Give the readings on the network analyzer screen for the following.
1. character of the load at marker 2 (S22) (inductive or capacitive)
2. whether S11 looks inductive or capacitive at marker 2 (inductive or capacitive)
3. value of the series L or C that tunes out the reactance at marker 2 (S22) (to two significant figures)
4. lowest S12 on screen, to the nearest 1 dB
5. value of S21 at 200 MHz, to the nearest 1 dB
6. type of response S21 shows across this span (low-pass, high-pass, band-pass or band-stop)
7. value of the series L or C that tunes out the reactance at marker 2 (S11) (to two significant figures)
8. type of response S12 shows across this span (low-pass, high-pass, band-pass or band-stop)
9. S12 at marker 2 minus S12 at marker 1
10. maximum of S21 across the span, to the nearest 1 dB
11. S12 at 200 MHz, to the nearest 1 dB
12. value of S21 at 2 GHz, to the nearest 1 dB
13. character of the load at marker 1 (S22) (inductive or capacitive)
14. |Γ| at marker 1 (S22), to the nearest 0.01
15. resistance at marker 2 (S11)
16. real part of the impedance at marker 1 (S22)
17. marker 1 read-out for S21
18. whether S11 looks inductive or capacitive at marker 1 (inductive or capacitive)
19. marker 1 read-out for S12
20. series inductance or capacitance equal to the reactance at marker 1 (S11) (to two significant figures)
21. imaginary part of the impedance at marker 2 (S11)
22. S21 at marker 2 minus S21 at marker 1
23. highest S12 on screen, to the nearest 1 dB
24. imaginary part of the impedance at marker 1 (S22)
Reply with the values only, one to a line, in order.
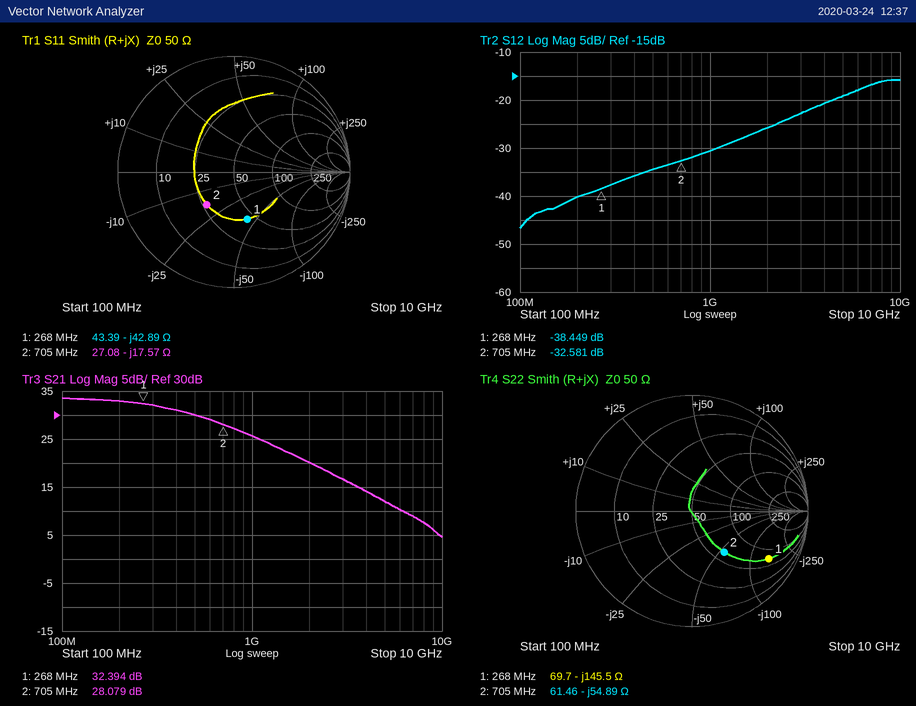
capacitive
capacitive
12 nH
-47 dB
33 dB
low-pass
4.0 nH
high-pass
5.868 dB
34 dB
-40 dB
20 dB
capacitive
0.78
27.08 Ω
69.7 Ω
32.394 dB
capacitive
-38.449 dB
14 pF
-17.57 Ω
-4.315 dB
-16 dB
-145.5 Ω
